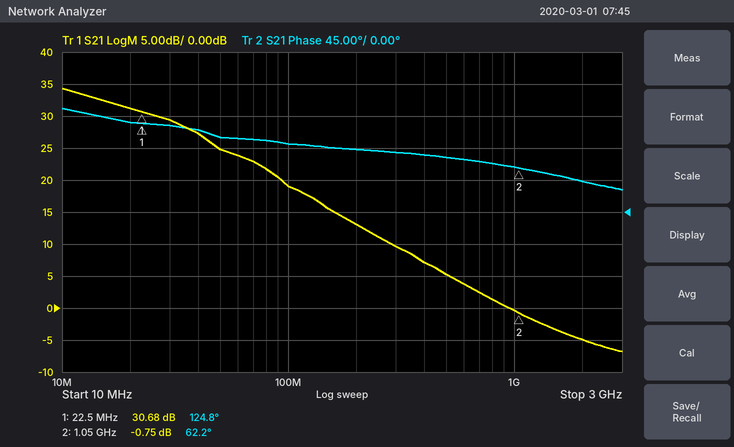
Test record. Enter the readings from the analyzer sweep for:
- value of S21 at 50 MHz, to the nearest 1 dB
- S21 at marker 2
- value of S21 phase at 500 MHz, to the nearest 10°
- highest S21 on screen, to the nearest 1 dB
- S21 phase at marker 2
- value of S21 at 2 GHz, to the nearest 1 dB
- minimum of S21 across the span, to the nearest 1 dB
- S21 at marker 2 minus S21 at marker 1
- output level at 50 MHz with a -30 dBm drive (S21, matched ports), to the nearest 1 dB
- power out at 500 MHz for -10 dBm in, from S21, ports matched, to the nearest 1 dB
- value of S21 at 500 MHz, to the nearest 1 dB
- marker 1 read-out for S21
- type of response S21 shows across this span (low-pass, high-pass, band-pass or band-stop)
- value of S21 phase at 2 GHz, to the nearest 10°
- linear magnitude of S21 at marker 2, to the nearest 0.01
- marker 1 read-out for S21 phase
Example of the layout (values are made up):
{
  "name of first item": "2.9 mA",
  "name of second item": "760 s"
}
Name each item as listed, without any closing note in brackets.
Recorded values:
{
  "value of S21 at 50 MHz, to the nearest 1 dB": "25 dB",
  "S21 at marker 2": "-0.75 dB",
  "value of S21 phase at 500 MHz, to the nearest 10°": "80°",
  "highest S21 on screen, to the nearest 1 dB": "34 dB",
  "S21 phase at marker 2": "62.2°",
  "value of S21 at 2 GHz, to the nearest 1 dB": "-5 dB",
  "minimum of S21 across the span, to the nearest 1 dB": "-7 dB",
  "S21 at marker 2 minus S21 at marker 1": "-31.43 dB",
  "output level at 50 MHz with a -30 dBm drive (S21, matched ports), to the nearest 1 dB": "-5 dBm",
  "power out at 500 MHz for -10 dBm in, from S21, ports matched, to the nearest 1 dB": "-5 dBm",
  "value of S21 at 500 MHz, to the nearest 1 dB": "5 dB",
  "marker 1 read-out for S21": "30.68 dB",
  "type of response S21 shows across this span": "low-pass",
  "value of S21 phase at 2 GHz, to the nearest 10°": "40°",
  "linear magnitude of S21 at marker 2, to the nearest 0.01": "0.92",
  "marker 1 read-out for S21 phase": "124.8°"
}
